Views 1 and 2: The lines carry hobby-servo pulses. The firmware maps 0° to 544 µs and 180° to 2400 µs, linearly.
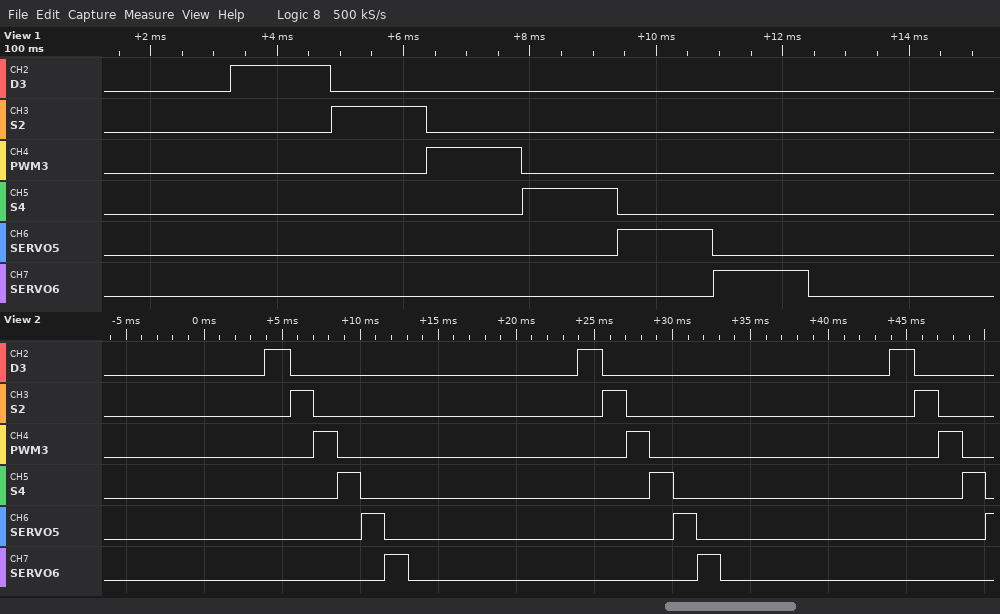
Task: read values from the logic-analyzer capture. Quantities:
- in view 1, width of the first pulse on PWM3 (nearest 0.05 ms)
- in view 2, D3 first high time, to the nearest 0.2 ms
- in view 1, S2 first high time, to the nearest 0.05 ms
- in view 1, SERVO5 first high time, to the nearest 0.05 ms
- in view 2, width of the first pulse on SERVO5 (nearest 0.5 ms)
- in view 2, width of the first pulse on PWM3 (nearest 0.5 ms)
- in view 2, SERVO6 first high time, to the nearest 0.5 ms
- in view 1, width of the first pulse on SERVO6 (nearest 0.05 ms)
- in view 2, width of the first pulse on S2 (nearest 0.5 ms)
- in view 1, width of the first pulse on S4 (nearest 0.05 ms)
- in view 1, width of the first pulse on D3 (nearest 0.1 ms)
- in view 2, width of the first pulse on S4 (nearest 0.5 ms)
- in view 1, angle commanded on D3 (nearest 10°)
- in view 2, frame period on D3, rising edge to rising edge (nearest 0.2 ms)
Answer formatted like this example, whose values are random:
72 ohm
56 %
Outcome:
1.50 ms
1.6 ms
1.50 ms
1.50 ms
1.5 ms
1.5 ms
1.5 ms
1.50 ms
1.5 ms
1.50 ms
1.6 ms
1.5 ms
100°
20.0 ms
